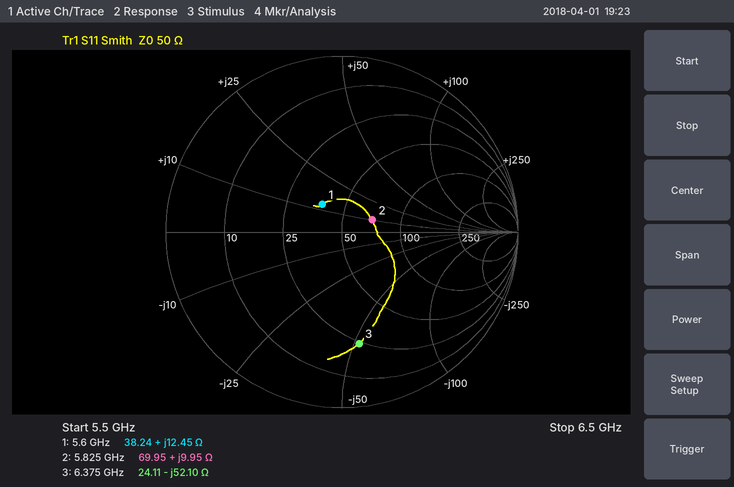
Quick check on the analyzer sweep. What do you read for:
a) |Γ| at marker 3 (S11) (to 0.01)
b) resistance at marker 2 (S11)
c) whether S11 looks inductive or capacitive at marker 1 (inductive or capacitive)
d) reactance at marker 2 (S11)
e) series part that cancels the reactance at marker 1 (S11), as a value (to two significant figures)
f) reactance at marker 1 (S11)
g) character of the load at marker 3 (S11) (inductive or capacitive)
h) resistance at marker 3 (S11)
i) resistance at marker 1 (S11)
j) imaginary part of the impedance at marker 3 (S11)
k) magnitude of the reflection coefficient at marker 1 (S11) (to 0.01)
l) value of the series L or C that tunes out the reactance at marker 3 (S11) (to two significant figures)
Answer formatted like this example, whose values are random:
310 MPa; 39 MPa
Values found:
0.64; 69.95 Ω; inductive; +9.95 Ω; 2.3 pF; +12.45 Ω; capacitive; 24.11 Ω; 38.24 Ω; -52.10 Ω; 0.19; 1.3 nH
